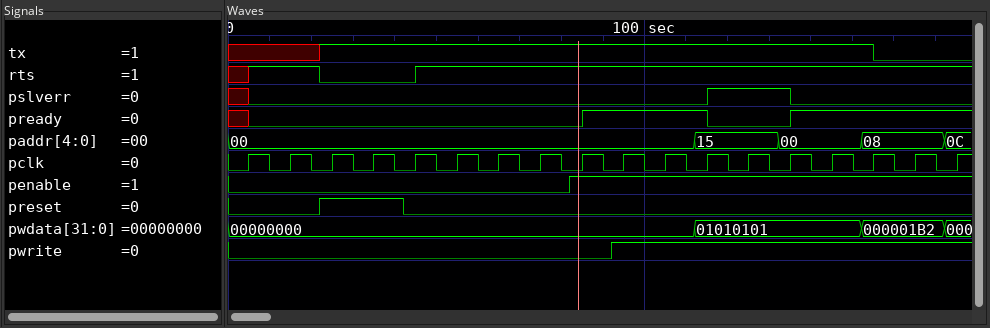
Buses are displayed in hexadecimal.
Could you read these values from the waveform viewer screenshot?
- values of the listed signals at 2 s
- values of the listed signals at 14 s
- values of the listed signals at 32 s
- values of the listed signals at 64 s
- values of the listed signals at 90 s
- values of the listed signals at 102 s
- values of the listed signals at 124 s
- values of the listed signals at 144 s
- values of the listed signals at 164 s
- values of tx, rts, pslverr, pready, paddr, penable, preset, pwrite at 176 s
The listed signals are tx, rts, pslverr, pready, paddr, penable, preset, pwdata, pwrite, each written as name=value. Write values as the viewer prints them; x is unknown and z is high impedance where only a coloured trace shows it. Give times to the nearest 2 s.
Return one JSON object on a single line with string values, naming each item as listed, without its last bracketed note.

{"values of the listed signals at 2 s": "tx=x, rts=x, pslverr=x, pready=x, paddr=00, penable=0, preset=0, pwdata=00000000, pwrite=0", "values of the listed signals at 14 s": "tx=x, rts=1, pslverr=0, pready=0, paddr=00, penable=0, preset=0, pwdata=00000000, pwrite=0", "values of the listed signals at 32 s": "tx=1, rts=0, pslverr=0, pready=0, paddr=00, penable=0, preset=1, pwdata=00000000, pwrite=0", "values of the listed signals at 64 s": "tx=1, rts=1, pslverr=0, pready=0, paddr=00, penable=0, preset=0, pwdata=00000000, pwrite=0", "values of the listed signals at 90 s": "tx=1, rts=1, pslverr=0, pready=1, paddr=00, penable=1, preset=0, pwdata=00000000, pwrite=0", "values of the listed signals at 102 s": "tx=1, rts=1, pslverr=0, pready=1, paddr=00, penable=1, preset=0, pwdata=00000000, pwrite=1", "values of the listed signals at 124 s": "tx=1, rts=1, pslverr=1, pready=0, paddr=15, penable=1, preset=0, pwdata=01010101, pwrite=1", "values of the listed signals at 144 s": "tx=1, rts=1, pslverr=0, pready=1, paddr=00, penable=1, preset=0, pwdata=01010101, pwrite=1", "values of the listed signals at 164 s": "tx=0, rts=1, pslverr=0, pready=1, paddr=08, penable=1, preset=0, pwdata=000001B2, pwrite=1", "values of tx, rts, pslverr, pready, paddr, penable, preset, pwrite at 176 s": "tx=0, rts=1, pslverr=0, pready=1, paddr=0C, penable=1, preset=0, pwrite=1"}
